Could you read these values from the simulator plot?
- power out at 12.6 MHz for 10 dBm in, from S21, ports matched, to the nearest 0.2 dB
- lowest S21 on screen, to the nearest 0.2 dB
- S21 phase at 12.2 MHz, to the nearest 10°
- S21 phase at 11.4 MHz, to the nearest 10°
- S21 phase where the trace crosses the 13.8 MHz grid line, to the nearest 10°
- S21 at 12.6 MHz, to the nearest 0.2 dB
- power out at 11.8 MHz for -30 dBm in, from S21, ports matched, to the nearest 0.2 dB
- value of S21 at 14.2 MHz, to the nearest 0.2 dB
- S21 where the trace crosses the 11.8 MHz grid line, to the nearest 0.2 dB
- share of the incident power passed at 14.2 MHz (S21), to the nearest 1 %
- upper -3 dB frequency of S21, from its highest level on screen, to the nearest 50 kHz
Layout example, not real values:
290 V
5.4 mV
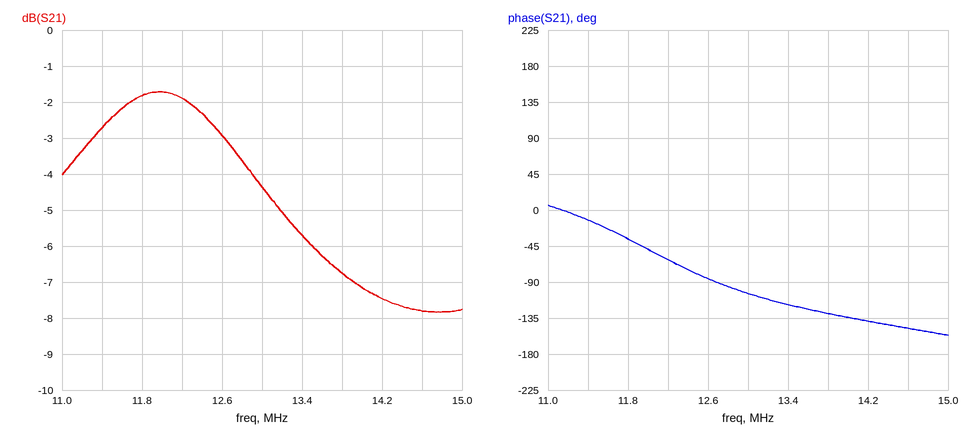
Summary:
7.0 dBm
-7.8 dB
-60°
-10°
-130°
-3.0 dB
-31.8 dBm
-7.4 dB
-1.8 dB
18 %
13.10 MHz
